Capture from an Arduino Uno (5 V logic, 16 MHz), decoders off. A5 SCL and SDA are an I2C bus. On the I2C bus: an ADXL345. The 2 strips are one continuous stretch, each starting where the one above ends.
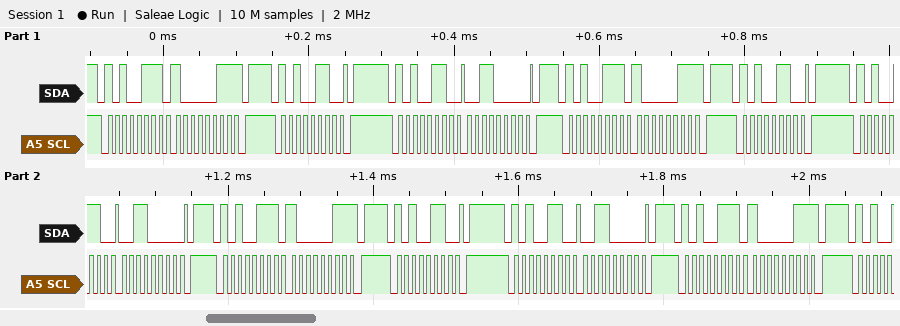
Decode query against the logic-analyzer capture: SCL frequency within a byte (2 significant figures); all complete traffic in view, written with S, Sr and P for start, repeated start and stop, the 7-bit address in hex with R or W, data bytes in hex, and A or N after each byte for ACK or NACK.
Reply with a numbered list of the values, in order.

1. 100 kHz
2. S 53R A 83 N P S 53W A P S 53W A 30 A P S 53R A 83 N P S 53W A P S 53W A 30 A P S 53R A 83 N P S 53W A P S 53W A 30 A P S 53R A 83 N P
